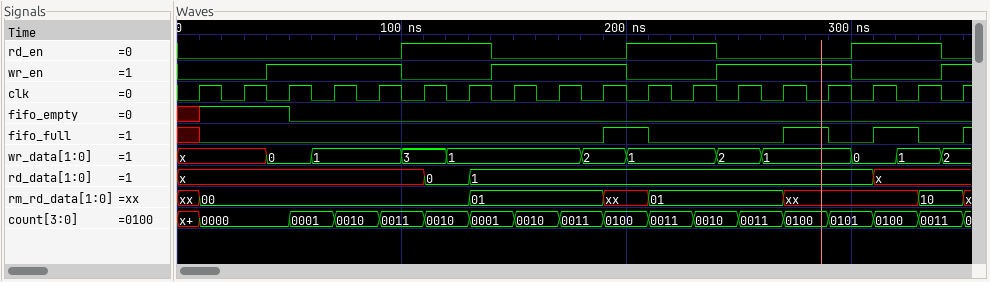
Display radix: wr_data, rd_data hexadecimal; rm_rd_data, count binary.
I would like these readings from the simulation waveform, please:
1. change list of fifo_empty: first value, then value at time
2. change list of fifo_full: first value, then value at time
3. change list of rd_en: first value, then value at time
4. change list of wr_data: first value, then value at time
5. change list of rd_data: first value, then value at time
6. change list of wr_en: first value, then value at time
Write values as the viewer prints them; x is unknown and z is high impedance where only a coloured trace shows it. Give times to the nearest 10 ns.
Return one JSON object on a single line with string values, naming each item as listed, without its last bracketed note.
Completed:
{"change list of fifo_empty: first value, then value at time": "x, 1 at 10 ns, 0 at 50 ns", "change list of fifo_full: first value, then value at time": "x, 0 at 10 ns, 1 at 190 ns, 0 at 210 ns, 1 at 270 ns, 0 at 290 ns, 1 at 310 ns, 0 at 330 ns, 1 at 350 ns", "change list of rd_en: first value, then value at time": "0, 1 at 100 ns, 0 at 140 ns, 1 at 200 ns, 0 at 240 ns, 1 at 300 ns, 0 at 340 ns", "change list of wr_data: first value, then value at time": "x, 0 at 40 ns, 1 at 60 ns, 3 at 100 ns, 1 at 120 ns, 2 at 180 ns, 1 at 200 ns, 2 at 240 ns, 1 at 260 ns, 0 at 300 ns, 1 at 320 ns, 2 at 340 ns", "change list of rd_data: first value, then value at time": "x, 0 at 110 ns, 1 at 130 ns, x at 310 ns", "change list of wr_en: first value, then value at time": "0, 1 at 40 ns, 0 at 100 ns, 1 at 140 ns, 0 at 200 ns, 1 at 240 ns, 0 at 300 ns, 1 at 340 ns"}
